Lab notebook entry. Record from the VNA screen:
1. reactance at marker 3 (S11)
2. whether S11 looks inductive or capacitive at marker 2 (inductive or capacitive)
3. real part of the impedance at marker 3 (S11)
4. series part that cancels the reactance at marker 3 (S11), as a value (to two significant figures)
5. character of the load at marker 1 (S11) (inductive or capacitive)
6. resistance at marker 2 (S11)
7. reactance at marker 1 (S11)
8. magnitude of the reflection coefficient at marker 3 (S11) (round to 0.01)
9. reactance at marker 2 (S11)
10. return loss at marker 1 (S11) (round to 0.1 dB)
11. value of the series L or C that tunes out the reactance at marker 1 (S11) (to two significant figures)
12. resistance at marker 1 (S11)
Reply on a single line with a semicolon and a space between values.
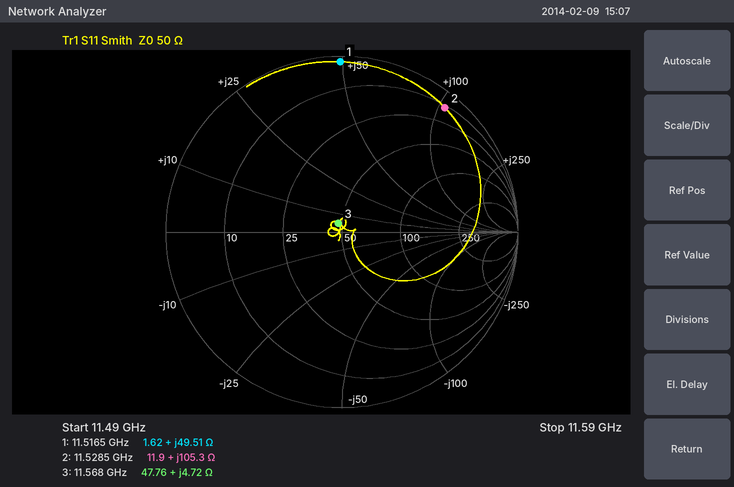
+4.72 Ω; inductive; 47.76 Ω; 2.9 pF; inductive; 11.9 Ω; +49.51 Ω; 0.05; +105.3 Ω; 0.3 dB; 280 fF; 1.62 Ω
